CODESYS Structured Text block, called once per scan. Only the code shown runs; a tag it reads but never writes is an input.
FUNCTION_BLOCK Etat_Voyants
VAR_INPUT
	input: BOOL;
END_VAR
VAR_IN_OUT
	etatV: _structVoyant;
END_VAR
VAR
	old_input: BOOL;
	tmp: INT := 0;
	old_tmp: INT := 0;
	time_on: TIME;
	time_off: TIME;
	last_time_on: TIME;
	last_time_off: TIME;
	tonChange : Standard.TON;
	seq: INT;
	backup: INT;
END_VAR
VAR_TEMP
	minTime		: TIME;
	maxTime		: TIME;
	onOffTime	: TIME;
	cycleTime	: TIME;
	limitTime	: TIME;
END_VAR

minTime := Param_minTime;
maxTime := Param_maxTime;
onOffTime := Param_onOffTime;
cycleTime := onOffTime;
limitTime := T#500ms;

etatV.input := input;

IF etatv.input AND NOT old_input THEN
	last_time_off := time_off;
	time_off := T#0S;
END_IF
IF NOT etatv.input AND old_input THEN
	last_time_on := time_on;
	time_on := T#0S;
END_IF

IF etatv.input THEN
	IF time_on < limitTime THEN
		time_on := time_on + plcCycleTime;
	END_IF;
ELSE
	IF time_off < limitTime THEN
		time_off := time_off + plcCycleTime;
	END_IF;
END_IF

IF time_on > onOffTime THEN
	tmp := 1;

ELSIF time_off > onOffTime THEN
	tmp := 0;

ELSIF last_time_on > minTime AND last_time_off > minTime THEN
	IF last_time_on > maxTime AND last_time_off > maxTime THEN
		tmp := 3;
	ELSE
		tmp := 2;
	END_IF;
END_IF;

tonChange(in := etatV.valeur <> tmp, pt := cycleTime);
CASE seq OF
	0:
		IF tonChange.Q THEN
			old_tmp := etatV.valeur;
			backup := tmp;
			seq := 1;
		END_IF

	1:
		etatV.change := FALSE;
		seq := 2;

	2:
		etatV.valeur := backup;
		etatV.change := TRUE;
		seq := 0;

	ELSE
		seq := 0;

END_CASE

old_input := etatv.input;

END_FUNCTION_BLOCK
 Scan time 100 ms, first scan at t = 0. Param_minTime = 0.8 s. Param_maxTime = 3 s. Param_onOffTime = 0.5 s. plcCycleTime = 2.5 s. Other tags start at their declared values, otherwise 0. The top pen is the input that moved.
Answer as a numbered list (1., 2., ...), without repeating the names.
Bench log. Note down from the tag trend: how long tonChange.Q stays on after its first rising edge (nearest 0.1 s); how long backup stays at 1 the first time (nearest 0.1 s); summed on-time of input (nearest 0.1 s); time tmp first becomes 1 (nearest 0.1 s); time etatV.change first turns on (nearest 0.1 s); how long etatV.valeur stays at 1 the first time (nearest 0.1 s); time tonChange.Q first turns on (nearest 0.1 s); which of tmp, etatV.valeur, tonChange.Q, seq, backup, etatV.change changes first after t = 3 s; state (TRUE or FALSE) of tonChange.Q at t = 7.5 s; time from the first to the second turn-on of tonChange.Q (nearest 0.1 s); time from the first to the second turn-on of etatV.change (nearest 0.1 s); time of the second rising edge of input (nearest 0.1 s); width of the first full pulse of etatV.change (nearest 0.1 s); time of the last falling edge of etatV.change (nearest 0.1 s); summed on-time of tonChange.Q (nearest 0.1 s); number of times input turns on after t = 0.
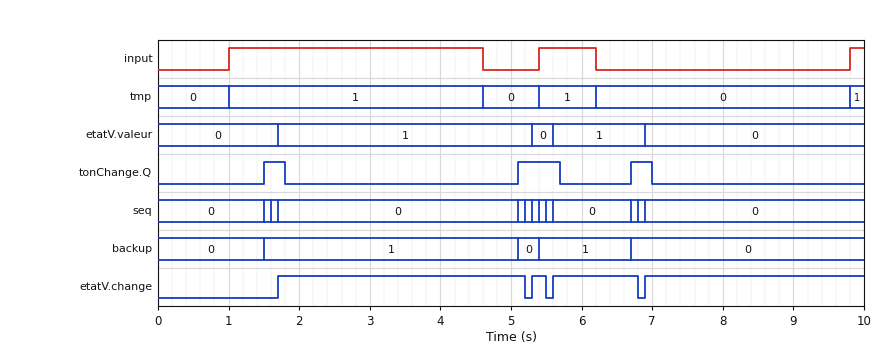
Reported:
1. 0.3 s
2. 3.6 s
3. 4.6 s
4. 1.0 s
5. 1.7 s
6. 3.6 s
7. 1.5 s
8. tmp
9. FALSE
10. 3.6 s
11. 3.6 s
12. 5.4 s
13. 3.5 s
14. 6.8 s
15. 1.2 s
16. 3
